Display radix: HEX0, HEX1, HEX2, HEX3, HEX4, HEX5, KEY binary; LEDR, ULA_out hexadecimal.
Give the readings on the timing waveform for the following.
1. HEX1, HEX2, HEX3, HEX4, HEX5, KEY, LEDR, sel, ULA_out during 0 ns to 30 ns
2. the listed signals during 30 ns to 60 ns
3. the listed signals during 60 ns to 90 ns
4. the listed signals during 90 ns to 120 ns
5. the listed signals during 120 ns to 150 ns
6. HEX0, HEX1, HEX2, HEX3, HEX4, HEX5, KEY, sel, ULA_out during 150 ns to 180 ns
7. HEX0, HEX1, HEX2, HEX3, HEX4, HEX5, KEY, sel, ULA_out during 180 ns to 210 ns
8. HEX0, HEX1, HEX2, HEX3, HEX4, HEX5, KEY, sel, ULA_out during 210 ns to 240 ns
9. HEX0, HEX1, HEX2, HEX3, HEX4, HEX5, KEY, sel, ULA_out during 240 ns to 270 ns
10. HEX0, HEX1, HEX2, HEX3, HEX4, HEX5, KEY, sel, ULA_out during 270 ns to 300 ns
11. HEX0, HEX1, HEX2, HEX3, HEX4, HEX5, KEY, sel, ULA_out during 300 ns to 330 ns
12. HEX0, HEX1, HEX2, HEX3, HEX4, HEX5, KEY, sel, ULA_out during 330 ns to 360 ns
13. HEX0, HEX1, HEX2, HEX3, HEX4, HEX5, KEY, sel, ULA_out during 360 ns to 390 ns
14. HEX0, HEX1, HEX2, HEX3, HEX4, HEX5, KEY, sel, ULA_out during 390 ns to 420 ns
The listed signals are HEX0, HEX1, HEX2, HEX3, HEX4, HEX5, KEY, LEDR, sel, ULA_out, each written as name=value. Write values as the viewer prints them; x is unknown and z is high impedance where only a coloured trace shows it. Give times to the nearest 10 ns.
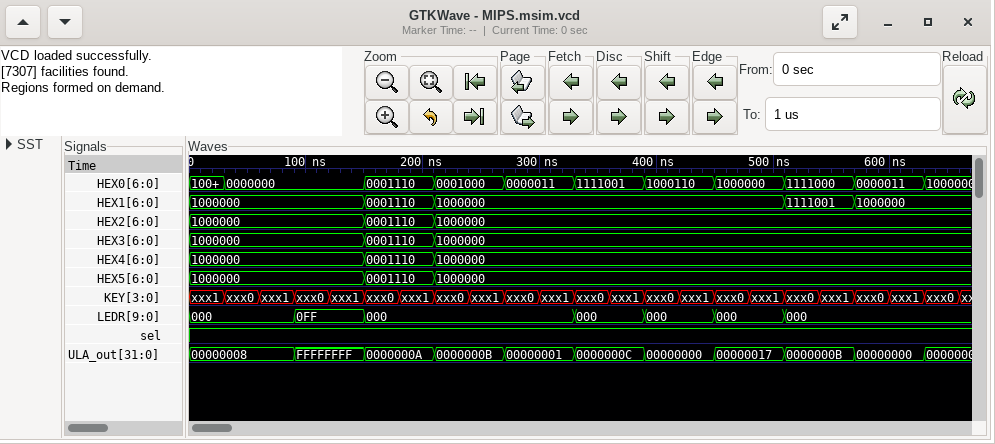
HEX1=1000000, HEX2=1000000, HEX3=1000000, HEX4=1000000, HEX5=1000000, KEY=xxx1, LEDR=000, sel=1, ULA_out=00000008
HEX0=0000000, HEX1=1000000, HEX2=1000000, HEX3=1000000, HEX4=1000000, HEX5=1000000, KEY=xxx0, LEDR=000, sel=1, ULA_out=00000008
HEX0=0000000, HEX1=1000000, HEX2=1000000, HEX3=1000000, HEX4=1000000, HEX5=1000000, KEY=xxx1, LEDR=000, sel=1, ULA_out=00000008
HEX0=0000000, HEX1=1000000, HEX2=1000000, HEX3=1000000, HEX4=1000000, HEX5=1000000, KEY=xxx0, LEDR=0FF, sel=1, ULA_out=FFFFFFFF
HEX0=0000000, HEX1=1000000, HEX2=1000000, HEX3=1000000, HEX4=1000000, HEX5=1000000, KEY=xxx1, LEDR=0FF, sel=1, ULA_out=FFFFFFFF
HEX0=0001110, HEX1=0001110, HEX2=0001110, HEX3=0001110, HEX4=0001110, HEX5=0001110, KEY=xxx0, sel=1, ULA_out=0000000A
HEX0=0001110, HEX1=0001110, HEX2=0001110, HEX3=0001110, HEX4=0001110, HEX5=0001110, KEY=xxx1, sel=1, ULA_out=0000000A
HEX0=0001000, HEX1=1000000, HEX2=1000000, HEX3=1000000, HEX4=1000000, HEX5=1000000, KEY=xxx0, sel=1, ULA_out=0000000B
HEX0=0001000, HEX1=1000000, HEX2=1000000, HEX3=1000000, HEX4=1000000, HEX5=1000000, KEY=xxx1, sel=1, ULA_out=0000000B
HEX0=0000011, HEX1=1000000, HEX2=1000000, HEX3=1000000, HEX4=1000000, HEX5=1000000, KEY=xxx0, sel=1, ULA_out=00000001
HEX0=0000011, HEX1=1000000, HEX2=1000000, HEX3=1000000, HEX4=1000000, HEX5=1000000, KEY=xxx1, sel=1, ULA_out=00000001
HEX0=1111001, HEX1=1000000, HEX2=1000000, HEX3=1000000, HEX4=1000000, HEX5=1000000, KEY=xxx0, sel=1, ULA_out=0000000C
HEX0=1111001, HEX1=1000000, HEX2=1000000, HEX3=1000000, HEX4=1000000, HEX5=1000000, KEY=xxx1, sel=1, ULA_out=0000000C
HEX0=1000110, HEX1=1000000, HEX2=1000000, HEX3=1000000, HEX4=1000000, HEX5=1000000, KEY=xxx0, sel=1, ULA_out=00000000
